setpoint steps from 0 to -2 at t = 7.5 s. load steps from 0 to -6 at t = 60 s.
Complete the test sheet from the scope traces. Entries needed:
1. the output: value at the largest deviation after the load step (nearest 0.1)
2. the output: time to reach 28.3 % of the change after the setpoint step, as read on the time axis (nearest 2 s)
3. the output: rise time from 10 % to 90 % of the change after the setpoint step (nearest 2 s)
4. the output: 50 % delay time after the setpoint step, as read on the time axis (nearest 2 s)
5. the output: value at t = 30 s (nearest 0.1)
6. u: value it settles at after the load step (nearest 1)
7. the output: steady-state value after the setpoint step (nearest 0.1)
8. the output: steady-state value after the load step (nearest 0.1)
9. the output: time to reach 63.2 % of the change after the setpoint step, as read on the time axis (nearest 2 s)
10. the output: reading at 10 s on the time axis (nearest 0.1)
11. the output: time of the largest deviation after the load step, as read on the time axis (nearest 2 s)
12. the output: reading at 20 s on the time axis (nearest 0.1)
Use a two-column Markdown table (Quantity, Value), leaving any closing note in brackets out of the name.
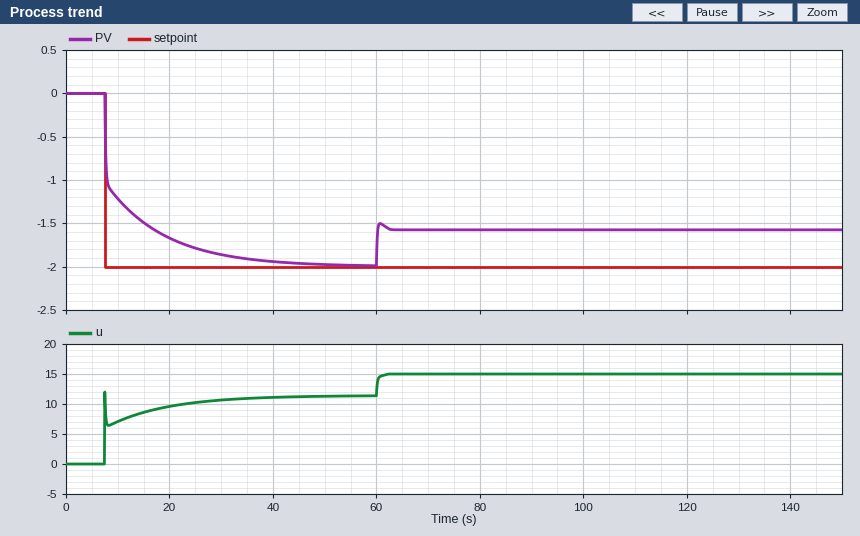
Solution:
| Quantity | Value |
|---|---|
| the output: value at the largest deviation after the load step | -1.5 |
| the output: time to reach 28.3 % of the change after the setpoint step, as read on the time axis | 8 s |
| the output: rise time from 10 % to 90 % of the change after the setpoint step | 18 s |
| the output: 50 % delay time after the setpoint step, as read on the time axis | 8 s |
| the output: value at t = 30 s | -1.9 |
| u: value it settles at after the load step | 15 |
| the output: steady-state value after the setpoint step | -2.0 |
| the output: steady-state value after the load step | -1.6 |
| the output: time to reach 63.2 % of the change after the setpoint step, as read on the time axis | 10 s |
| the output: reading at 10 s on the time axis | -1.2 |
| the output: time of the largest deviation after the load step, as read on the time axis | 60 s |
| the output: reading at 20 s on the time axis | -1.7 |
